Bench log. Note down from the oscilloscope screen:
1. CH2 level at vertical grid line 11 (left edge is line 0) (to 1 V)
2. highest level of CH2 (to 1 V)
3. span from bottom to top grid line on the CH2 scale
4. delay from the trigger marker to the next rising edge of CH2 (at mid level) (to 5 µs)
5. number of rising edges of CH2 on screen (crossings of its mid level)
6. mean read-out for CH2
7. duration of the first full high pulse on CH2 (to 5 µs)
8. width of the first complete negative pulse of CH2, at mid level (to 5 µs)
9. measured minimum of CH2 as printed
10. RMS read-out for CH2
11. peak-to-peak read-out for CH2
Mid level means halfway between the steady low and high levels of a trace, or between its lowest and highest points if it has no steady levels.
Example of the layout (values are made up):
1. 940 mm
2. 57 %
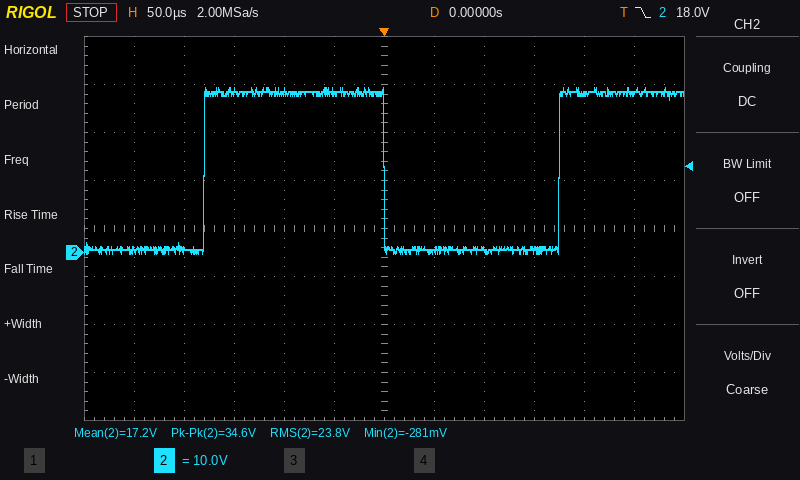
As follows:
1. 33 V
2. 34 V
3. 80 V
4. 175 µs
5. 2
6. 17.2 V
7. 180 µs
8. 175 µs
9. -281 mV
10. 23.8 V
11. 34.6 V
